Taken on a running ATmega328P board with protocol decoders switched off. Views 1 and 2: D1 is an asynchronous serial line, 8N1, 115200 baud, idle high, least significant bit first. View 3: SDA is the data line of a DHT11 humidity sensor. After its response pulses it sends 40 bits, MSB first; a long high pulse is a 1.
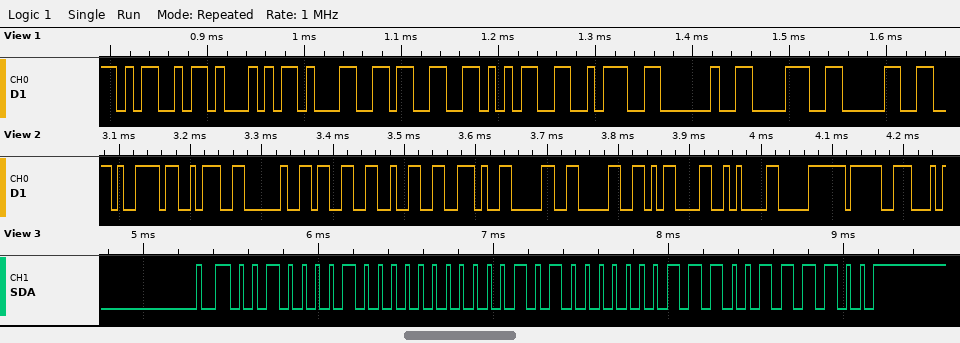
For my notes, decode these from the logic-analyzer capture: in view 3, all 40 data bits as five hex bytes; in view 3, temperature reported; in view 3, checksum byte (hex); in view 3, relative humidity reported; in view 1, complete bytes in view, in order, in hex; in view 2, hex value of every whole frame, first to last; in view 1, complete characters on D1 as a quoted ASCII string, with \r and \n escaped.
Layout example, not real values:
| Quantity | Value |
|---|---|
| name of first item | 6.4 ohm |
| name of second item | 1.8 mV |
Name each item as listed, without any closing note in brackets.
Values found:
| Quantity | Value |
|---|---|
| in view 3, all 40 data bits as five hex bytes | 21 00 14 07 3C |
| in view 3, temperature reported | 20.7 °C |
| in view 3, checksum byte | 0x3C |
| in view 3, relative humidity reported | 33 % |
| in view 1, complete bytes in view, in order, in hex | 4D 51 31 33 35 3A 20 38 30 |
| in view 2, hex value of every whole frame, first to last | 0x79 0x3A 0x20 0x33 0x32 0x2E 0x30 0x30 0x0D 0x0A 0xF0 0x9F |
| in view 1, complete characters on D1 as a quoted ASCII string, with \r and \n escaped | "MQ135: 80" |
